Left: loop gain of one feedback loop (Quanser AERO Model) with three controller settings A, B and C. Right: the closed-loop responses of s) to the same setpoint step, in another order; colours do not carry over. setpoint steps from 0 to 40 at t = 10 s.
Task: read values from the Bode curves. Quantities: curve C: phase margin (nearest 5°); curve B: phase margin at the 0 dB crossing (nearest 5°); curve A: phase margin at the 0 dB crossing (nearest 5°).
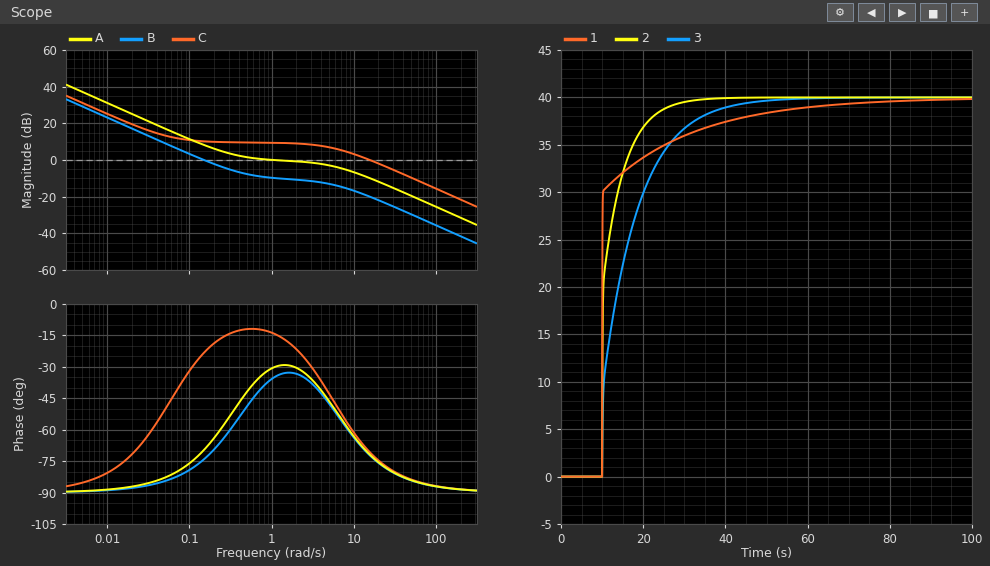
110°
105°
150°
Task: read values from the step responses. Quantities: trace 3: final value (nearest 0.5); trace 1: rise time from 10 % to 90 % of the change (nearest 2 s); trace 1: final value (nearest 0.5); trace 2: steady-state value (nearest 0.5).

40.0
20 s
40.0
40.0
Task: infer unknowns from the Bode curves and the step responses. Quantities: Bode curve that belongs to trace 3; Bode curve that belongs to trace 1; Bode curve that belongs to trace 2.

B
C
A
